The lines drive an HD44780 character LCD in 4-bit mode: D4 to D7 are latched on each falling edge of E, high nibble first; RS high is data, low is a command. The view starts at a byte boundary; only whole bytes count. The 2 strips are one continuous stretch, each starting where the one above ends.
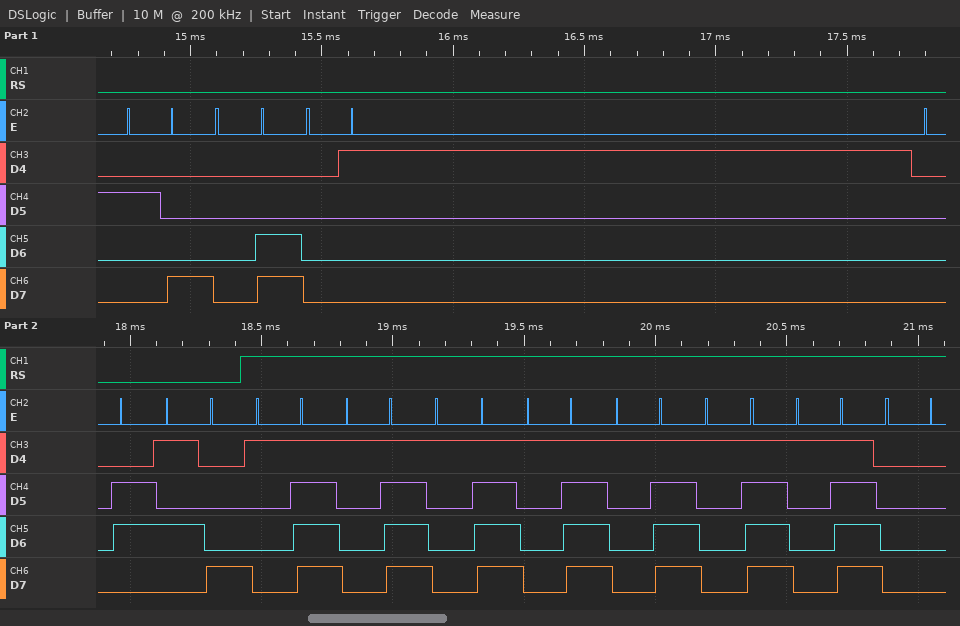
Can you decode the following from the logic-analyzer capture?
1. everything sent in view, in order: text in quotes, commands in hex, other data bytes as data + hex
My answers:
0x28 0x0C 0x01 0x06 0x58 data 1F 1F 1F 1F 1F 1F 1F 00
